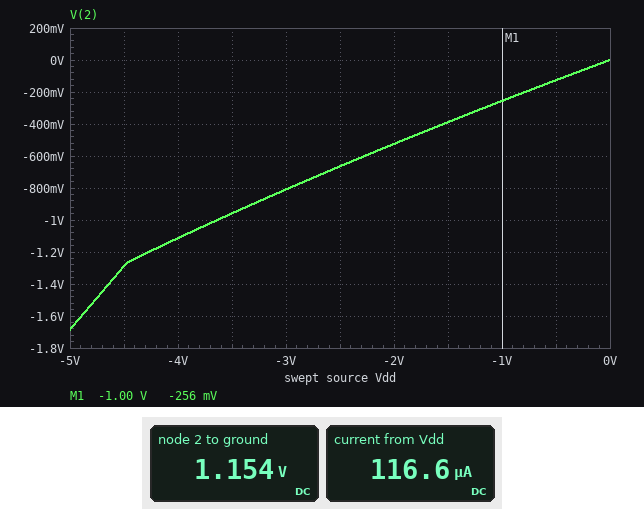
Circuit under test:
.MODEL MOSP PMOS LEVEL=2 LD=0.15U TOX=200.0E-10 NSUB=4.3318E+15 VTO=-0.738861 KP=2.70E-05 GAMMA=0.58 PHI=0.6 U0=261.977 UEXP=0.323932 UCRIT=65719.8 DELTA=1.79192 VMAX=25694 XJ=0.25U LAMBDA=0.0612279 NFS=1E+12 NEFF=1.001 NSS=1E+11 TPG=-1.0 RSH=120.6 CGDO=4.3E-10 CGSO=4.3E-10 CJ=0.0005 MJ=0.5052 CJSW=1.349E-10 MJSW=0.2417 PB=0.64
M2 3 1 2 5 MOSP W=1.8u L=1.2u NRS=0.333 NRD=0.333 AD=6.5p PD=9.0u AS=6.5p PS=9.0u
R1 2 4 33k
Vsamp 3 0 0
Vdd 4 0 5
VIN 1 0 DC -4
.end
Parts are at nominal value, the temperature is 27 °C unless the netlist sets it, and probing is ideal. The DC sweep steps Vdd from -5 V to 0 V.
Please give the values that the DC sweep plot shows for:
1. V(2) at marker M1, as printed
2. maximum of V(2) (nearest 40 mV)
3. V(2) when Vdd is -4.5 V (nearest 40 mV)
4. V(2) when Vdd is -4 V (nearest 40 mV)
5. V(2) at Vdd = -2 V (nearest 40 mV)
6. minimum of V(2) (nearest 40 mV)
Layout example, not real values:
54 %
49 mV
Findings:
-256 mV
0 V
-1.28 V
-1.12 V
-520 mV
-1.68 V
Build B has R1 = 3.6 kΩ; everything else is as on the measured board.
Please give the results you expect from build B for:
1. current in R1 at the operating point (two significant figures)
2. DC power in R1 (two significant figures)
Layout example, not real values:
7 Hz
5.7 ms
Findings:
320 µA
360 µW
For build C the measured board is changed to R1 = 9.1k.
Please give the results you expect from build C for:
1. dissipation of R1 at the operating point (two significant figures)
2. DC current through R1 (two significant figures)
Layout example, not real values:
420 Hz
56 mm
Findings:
530 µW
240 µA
